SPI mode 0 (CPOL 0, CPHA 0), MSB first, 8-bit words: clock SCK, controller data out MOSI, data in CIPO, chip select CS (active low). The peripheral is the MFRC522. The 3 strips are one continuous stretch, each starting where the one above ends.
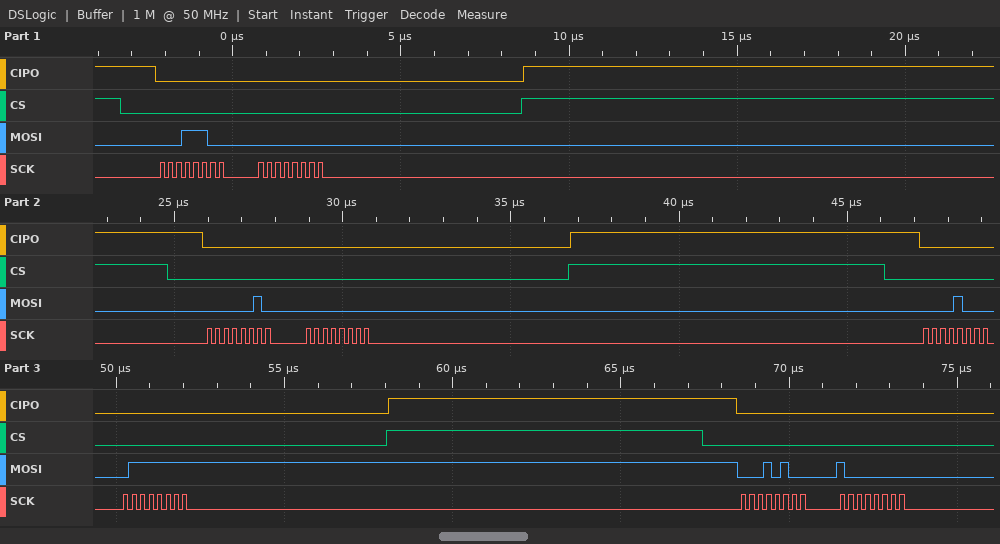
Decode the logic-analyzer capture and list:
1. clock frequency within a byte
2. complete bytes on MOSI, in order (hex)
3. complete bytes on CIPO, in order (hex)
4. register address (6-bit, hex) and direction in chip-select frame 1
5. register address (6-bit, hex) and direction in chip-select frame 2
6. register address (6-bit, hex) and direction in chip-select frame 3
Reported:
4 MHz
1C 00 02 00 08 7F 14 80
00 00 00 00 00 00 00 00
0x0E write
0x01 write
0x04 write
